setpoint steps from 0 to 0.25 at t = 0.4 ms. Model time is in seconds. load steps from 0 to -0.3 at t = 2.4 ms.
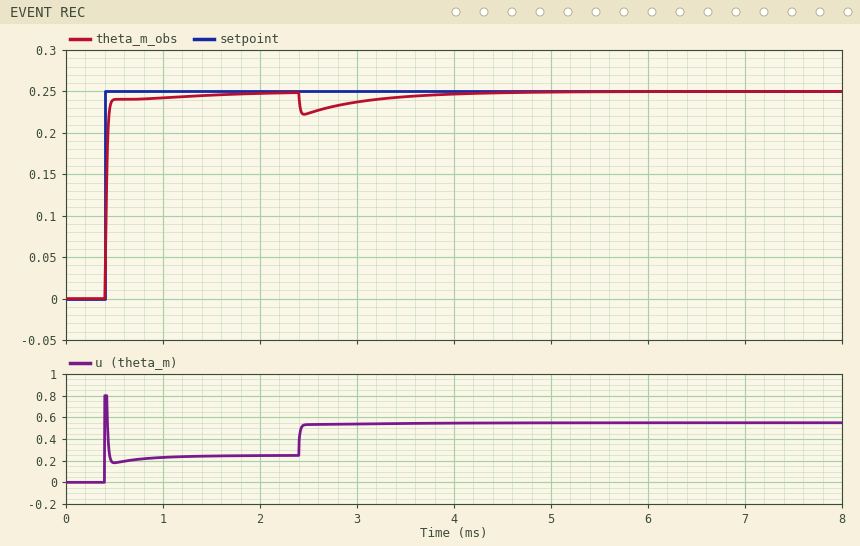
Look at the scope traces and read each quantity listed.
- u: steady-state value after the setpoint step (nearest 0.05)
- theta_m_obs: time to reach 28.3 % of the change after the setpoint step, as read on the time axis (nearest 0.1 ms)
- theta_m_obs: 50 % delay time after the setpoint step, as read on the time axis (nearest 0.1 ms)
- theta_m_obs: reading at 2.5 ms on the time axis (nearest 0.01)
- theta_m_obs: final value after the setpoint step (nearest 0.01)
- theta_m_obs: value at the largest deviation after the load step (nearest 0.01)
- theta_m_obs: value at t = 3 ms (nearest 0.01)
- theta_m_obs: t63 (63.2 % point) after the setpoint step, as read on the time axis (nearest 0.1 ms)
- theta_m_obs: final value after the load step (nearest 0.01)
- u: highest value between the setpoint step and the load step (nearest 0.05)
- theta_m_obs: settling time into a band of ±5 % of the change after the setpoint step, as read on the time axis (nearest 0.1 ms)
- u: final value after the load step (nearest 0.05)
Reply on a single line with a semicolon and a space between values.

0.25; 0.4 ms; 0.4 ms; 0.22; 0.25; 0.22; 0.24; 0.4 ms; 0.25; 0.80; 0.5 ms; 0.55
